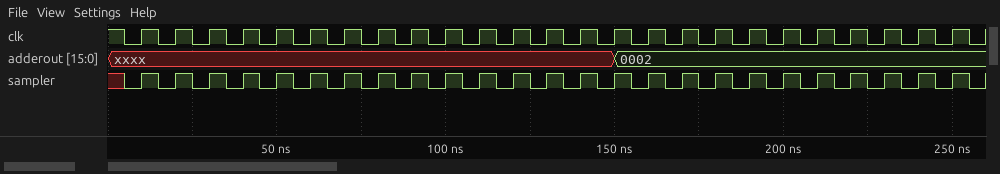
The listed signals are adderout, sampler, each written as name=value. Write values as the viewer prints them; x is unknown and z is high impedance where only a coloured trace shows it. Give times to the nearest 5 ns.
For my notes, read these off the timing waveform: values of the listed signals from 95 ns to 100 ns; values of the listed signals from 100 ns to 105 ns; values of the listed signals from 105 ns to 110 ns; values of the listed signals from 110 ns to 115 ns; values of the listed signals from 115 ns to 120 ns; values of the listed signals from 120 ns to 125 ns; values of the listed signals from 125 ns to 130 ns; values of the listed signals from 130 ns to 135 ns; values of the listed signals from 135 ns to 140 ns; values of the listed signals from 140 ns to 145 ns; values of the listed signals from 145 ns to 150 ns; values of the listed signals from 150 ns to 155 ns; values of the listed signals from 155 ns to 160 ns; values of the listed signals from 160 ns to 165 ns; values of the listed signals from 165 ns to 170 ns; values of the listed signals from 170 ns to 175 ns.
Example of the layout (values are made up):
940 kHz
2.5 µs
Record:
adderout=xxxx, sampler=0
adderout=xxxx, sampler=1
adderout=xxxx, sampler=0
adderout=xxxx, sampler=1
adderout=xxxx, sampler=0
adderout=xxxx, sampler=1
adderout=xxxx, sampler=0
adderout=xxxx, sampler=1
adderout=xxxx, sampler=0
adderout=xxxx, sampler=1
adderout=xxxx, sampler=0
adderout=0002, sampler=1
adderout=0002, sampler=0
adderout=0002, sampler=1
adderout=0002, sampler=0
adderout=0002, sampler=1
